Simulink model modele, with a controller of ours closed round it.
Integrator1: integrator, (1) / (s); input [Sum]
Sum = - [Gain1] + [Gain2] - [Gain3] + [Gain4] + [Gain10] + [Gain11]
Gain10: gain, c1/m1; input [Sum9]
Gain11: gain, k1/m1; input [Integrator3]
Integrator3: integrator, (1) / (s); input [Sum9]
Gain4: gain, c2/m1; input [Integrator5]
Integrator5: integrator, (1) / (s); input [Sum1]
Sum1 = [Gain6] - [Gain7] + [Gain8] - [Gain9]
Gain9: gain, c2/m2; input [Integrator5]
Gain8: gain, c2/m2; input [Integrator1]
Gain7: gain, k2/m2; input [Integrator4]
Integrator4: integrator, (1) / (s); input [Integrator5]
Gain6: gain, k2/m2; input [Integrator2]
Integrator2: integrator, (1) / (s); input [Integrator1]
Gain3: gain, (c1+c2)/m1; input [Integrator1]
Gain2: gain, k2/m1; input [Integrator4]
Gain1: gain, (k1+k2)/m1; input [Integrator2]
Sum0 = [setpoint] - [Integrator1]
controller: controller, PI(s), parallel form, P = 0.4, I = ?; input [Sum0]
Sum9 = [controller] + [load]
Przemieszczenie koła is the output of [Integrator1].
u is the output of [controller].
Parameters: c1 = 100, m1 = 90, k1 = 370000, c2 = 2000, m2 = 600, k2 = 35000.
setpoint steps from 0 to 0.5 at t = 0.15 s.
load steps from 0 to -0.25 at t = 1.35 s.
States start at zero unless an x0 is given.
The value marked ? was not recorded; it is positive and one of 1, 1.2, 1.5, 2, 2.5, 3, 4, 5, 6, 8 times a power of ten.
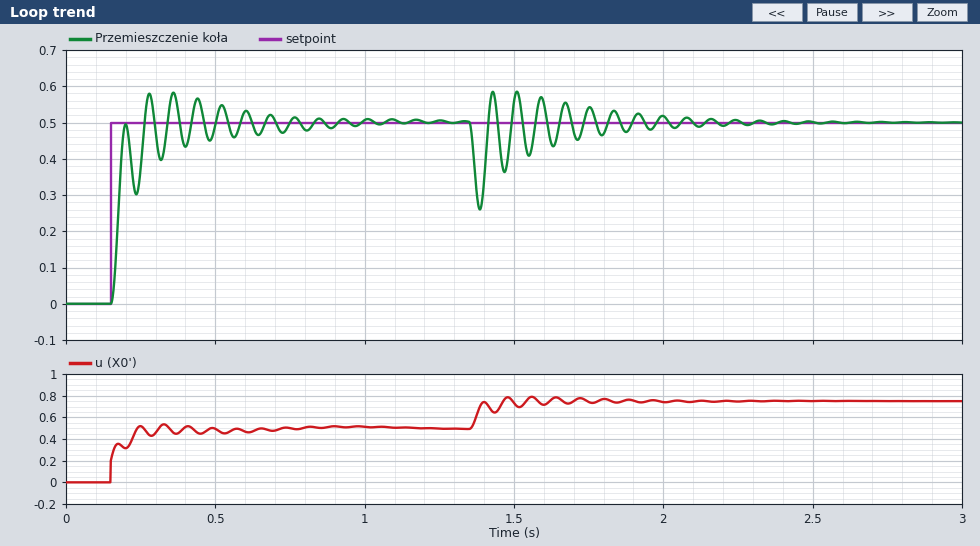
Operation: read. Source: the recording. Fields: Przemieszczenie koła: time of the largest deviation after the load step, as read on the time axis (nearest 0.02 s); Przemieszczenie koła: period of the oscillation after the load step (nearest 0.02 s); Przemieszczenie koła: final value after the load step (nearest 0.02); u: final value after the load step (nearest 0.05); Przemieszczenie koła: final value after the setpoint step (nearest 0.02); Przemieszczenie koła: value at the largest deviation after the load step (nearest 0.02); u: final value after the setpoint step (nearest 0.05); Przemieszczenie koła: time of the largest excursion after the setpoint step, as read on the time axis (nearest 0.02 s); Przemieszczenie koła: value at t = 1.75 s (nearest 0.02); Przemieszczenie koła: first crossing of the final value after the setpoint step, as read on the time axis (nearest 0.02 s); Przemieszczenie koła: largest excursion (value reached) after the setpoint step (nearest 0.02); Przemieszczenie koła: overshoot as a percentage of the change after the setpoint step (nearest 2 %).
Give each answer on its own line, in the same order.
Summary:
1.38 s
0.08 s
0.50
0.75
0.50
0.26
0.50
0.36 s
0.54
0.26 s
0.58
16 %
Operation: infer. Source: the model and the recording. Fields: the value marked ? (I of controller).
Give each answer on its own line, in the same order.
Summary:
25
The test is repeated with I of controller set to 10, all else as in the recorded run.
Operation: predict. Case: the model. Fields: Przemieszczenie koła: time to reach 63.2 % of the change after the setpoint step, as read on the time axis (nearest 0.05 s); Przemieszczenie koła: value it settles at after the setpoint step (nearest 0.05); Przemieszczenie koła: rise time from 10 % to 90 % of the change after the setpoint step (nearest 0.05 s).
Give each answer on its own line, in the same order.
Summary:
0.20 s
0.50
0.20 s
